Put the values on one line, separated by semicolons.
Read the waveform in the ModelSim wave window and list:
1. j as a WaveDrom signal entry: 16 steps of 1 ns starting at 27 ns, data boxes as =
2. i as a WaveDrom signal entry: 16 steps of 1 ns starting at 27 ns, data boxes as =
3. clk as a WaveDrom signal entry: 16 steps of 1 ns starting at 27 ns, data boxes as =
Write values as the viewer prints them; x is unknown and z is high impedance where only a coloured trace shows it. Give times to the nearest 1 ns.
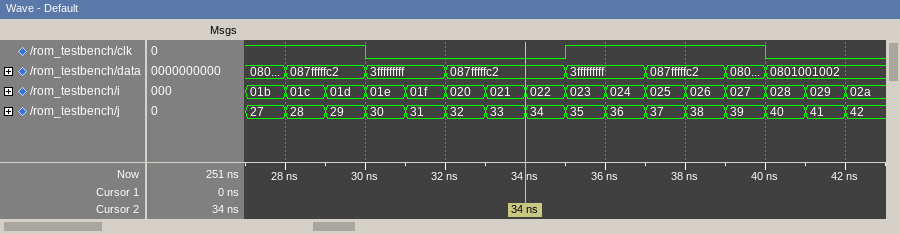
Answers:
{name: 'j', wave: '================', data: '27 28 29 30 31 32 33 34 35 36 37 38 39 40 41 42'}; {name: 'i', wave: '================', data: '01b 01c 01d 01e 01f 020 021 022 023 024 025 026 027 028 029 02a'}; {name: 'clk', wave: '1..0....1....0..'}
